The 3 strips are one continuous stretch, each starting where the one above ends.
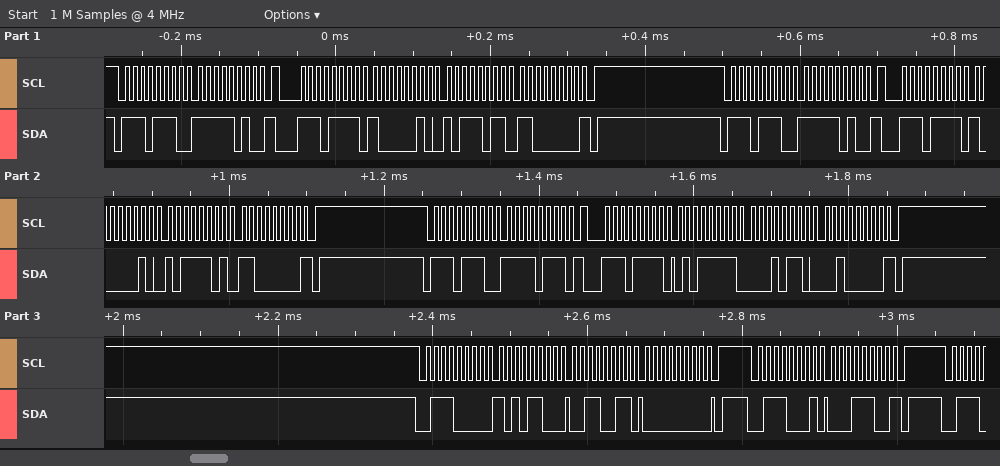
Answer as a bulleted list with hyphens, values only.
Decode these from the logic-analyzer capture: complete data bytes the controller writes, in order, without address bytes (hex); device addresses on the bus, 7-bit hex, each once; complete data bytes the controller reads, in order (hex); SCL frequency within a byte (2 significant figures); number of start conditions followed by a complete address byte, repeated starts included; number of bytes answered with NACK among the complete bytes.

- FA FA F7 AC 33 00
- 0x77 0x38
- 82 BB C0 82 BD C0 5F 16 20 1C
- 100 kHz
- 8
- 4
